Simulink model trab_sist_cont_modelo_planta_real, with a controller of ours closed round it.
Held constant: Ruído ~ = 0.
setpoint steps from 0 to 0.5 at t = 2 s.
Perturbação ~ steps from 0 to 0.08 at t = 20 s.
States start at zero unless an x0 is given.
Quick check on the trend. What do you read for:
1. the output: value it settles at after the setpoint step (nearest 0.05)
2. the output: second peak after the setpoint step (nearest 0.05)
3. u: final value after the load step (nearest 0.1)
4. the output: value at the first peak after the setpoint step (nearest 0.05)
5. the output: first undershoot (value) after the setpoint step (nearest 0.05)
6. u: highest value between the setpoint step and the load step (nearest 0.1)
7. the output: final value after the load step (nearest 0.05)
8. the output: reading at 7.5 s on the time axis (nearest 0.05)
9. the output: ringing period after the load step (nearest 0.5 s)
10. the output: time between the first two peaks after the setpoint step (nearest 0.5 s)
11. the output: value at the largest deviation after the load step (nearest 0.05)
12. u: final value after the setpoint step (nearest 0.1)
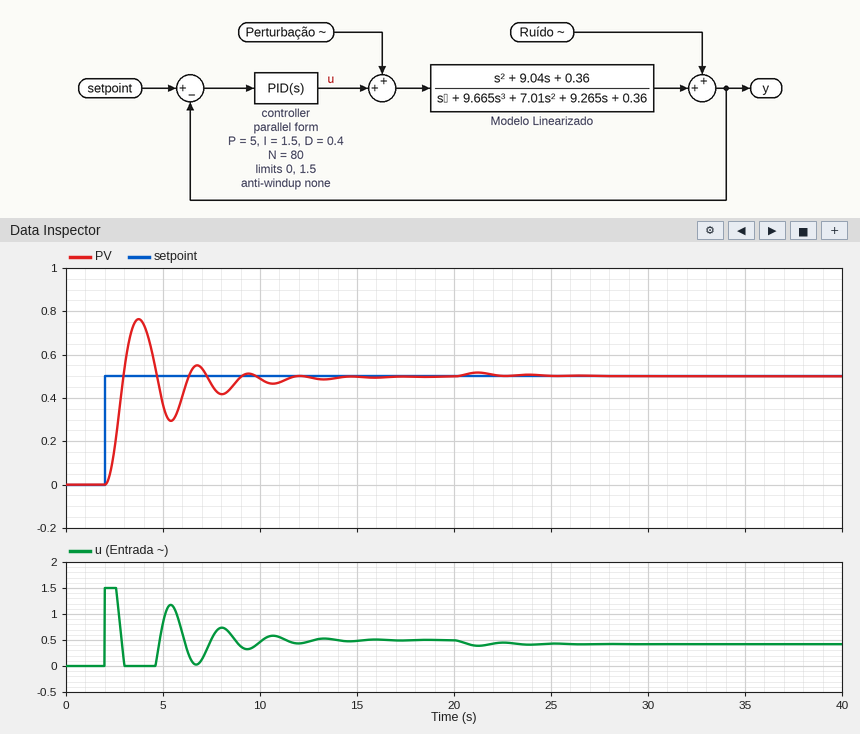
0.50
0.55
0.4
0.75
0.30
1.5
0.50
0.45
2.5 s
3.0 s
0.50
0.5
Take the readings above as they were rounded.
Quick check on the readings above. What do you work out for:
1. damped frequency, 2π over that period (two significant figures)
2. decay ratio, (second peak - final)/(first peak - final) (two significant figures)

2.1 rad/s
0.20
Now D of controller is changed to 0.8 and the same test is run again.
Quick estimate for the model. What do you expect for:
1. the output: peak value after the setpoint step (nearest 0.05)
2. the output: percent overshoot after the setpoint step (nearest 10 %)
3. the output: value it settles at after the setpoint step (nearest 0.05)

0.70
40 %
0.50
